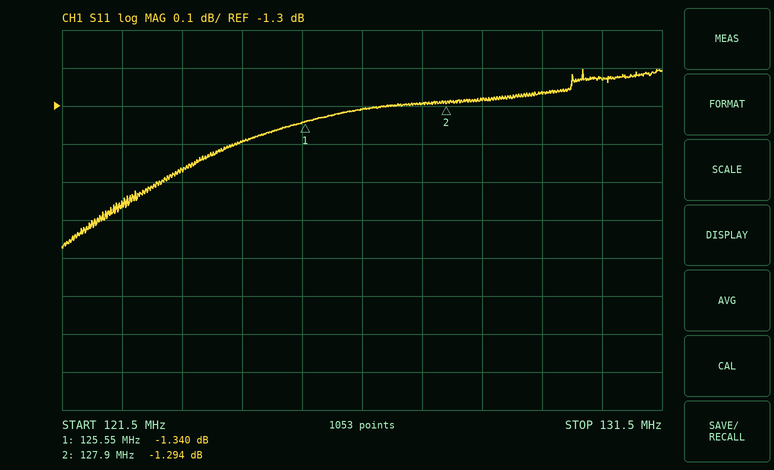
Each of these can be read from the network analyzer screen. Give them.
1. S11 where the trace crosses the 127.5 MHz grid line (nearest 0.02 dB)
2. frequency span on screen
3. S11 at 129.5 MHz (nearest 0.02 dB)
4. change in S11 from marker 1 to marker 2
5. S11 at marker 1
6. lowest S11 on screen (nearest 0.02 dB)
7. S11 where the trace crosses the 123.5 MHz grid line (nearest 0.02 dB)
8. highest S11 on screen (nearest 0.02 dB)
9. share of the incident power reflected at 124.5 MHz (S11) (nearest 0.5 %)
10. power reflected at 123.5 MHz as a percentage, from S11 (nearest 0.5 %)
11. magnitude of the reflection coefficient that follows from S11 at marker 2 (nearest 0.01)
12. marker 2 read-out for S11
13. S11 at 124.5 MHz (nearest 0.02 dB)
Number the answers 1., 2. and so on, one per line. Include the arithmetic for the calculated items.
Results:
1. -1.30 dB
2. 10 MHz
3. -1.26 dB
4. -1.294 − (-1.34) = 0.046 dB
5. -1.340 dB
6. -1.68 dB
7. -1.46 dB
8. -1.20 dB
9. 10^(-1.4/10) ≈ 72.4 %, so 72.5 % to the nearest 0.5 %
10. 10^(-1.46/10) ≈ 71.4 %, so 71.5 % to the nearest 0.5 %
11. 10^(-1.294/20) ≈ 0.86
12. -1.294 dB
13. -1.40 dB
